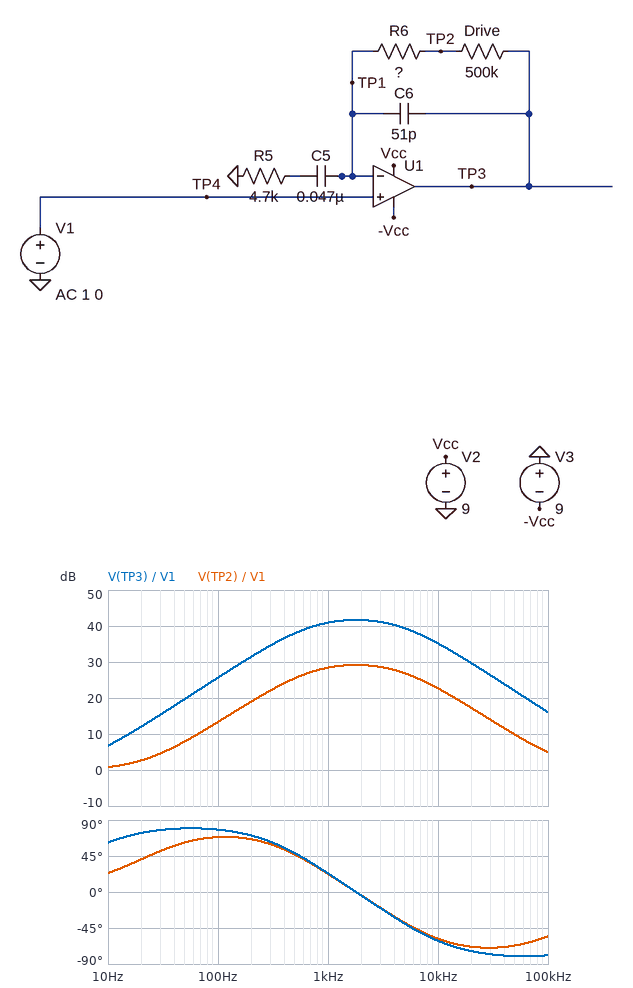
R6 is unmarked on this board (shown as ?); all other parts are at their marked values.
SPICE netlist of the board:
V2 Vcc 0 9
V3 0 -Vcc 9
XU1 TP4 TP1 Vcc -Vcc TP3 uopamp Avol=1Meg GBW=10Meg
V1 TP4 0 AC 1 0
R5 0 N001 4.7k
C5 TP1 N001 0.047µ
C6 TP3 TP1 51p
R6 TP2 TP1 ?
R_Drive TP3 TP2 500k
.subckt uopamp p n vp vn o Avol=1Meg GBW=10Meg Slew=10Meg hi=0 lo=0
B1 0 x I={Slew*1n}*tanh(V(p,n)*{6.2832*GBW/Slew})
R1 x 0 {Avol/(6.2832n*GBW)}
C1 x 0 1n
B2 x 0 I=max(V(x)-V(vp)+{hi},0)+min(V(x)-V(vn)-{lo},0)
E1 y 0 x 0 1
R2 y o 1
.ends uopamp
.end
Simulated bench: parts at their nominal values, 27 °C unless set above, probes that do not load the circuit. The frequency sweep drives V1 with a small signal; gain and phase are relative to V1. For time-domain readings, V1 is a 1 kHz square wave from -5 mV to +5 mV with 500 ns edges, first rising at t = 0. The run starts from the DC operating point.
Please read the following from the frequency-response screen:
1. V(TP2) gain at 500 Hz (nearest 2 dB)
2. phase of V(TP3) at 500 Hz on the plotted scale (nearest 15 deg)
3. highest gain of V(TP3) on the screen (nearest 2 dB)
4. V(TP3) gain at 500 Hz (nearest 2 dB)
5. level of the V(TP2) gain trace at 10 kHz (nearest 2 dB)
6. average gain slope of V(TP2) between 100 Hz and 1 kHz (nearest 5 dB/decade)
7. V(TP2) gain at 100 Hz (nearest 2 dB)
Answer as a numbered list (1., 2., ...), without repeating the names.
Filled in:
1. 26 dB
2. 45 deg
3. 42 dB
4. 38 dB
5. 22 dB
6. 15 dB/decade
7. 14 dB
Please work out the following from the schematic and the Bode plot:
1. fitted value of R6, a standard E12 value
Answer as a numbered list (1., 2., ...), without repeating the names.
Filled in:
1. 150 kΩ
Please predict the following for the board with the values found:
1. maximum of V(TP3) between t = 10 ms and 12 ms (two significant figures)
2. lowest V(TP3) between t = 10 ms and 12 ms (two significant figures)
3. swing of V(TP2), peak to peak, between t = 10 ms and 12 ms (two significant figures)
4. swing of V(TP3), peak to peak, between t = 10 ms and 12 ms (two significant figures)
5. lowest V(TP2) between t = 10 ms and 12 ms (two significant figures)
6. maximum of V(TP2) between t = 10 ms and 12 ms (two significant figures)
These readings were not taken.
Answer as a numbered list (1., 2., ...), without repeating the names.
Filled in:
1. 880 mV
2. -880 mV
3. 410 mV
4. 1.8 V
5. -210 mV
6. 210 mV
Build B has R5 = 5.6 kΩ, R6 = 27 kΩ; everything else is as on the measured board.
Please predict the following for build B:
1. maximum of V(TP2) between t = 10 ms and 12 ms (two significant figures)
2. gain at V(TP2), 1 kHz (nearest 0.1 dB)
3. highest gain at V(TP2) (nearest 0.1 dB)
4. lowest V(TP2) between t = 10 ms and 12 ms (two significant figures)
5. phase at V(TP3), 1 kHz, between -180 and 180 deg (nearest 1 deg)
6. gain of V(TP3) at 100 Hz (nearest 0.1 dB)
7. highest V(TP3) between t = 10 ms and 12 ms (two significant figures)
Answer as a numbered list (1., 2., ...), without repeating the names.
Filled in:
1. 37 mV
2. 14.0 dB
3. 14.6 dB
4. -37 mV
5. 21 deg
6. 23.8 dB
7. 620 mV
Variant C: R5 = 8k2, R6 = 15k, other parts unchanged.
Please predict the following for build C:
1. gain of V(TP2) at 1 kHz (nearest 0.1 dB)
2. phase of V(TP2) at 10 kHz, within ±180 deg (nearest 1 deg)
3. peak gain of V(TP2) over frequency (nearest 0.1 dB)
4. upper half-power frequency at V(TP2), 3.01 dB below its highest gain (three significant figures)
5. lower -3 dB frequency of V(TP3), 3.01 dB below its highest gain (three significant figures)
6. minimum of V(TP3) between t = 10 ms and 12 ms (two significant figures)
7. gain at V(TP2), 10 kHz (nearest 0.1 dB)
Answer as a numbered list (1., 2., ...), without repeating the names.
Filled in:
1. 8.5 dB
2. -28 deg
3. 8.7 dB
4. 7.53 kHz
5. 365 Hz
6. -400 mV
7. 4.5 dB
